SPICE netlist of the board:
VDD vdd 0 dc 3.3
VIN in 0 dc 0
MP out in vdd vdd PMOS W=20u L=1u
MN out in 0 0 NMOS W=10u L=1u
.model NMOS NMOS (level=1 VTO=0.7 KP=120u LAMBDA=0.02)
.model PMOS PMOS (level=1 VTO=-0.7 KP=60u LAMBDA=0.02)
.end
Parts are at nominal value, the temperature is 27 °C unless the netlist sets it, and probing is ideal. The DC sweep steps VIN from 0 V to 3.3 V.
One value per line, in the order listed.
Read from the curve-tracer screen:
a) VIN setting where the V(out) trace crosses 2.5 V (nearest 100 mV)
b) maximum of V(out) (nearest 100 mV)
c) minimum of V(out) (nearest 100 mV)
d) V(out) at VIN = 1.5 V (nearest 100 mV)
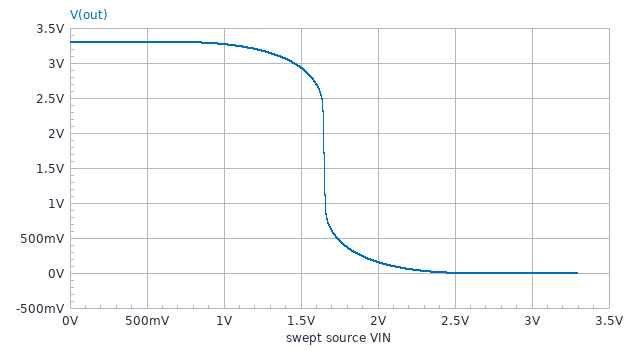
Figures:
1.6 V
3.3 V
0 V
2.9 V
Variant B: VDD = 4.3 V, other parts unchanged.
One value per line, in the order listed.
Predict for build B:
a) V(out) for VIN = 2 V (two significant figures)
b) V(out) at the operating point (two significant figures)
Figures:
3.6 V
4.3 V
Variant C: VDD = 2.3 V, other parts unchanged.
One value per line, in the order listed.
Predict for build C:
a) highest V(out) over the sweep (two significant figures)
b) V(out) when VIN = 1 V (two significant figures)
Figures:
2.3 V
2.2 V
